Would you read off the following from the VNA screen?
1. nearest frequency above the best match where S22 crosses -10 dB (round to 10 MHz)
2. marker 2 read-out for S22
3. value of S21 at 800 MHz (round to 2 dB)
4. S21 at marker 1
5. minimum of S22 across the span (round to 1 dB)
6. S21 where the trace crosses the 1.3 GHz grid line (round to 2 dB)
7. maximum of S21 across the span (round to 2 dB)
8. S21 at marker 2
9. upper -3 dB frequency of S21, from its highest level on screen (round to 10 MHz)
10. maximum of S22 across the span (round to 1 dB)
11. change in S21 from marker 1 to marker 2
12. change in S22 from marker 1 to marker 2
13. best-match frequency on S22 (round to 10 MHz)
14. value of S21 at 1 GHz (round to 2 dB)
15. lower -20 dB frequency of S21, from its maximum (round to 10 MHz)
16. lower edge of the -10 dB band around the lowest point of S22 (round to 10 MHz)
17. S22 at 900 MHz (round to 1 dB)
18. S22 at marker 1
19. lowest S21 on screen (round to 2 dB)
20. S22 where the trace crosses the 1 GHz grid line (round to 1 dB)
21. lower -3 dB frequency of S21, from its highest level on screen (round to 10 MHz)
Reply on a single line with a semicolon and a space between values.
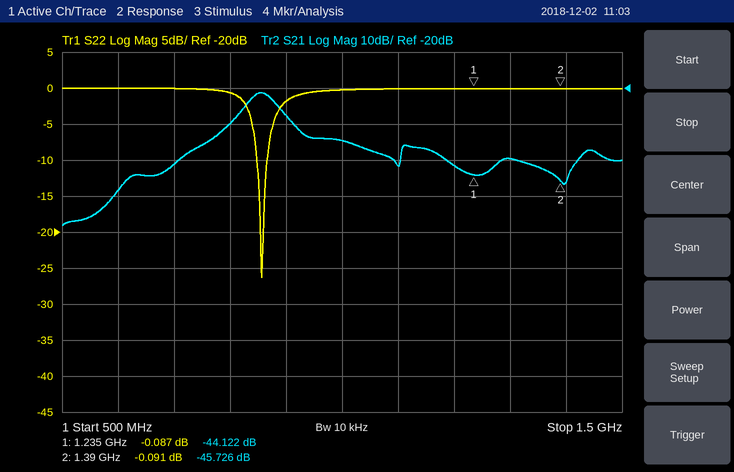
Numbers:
870 MHz; -0.091 dB; -30 dB; -44.122 dB; -26 dB; -40 dB; -22 dB; -45.726 dB; 880 MHz; 0 dB; -1.604 dB; -0.004 dB; 860 MHz; -34 dB; 700 MHz; 850 MHz; -2 dB; -0.087 dB; -58 dB; 0 dB; 830 MHz
